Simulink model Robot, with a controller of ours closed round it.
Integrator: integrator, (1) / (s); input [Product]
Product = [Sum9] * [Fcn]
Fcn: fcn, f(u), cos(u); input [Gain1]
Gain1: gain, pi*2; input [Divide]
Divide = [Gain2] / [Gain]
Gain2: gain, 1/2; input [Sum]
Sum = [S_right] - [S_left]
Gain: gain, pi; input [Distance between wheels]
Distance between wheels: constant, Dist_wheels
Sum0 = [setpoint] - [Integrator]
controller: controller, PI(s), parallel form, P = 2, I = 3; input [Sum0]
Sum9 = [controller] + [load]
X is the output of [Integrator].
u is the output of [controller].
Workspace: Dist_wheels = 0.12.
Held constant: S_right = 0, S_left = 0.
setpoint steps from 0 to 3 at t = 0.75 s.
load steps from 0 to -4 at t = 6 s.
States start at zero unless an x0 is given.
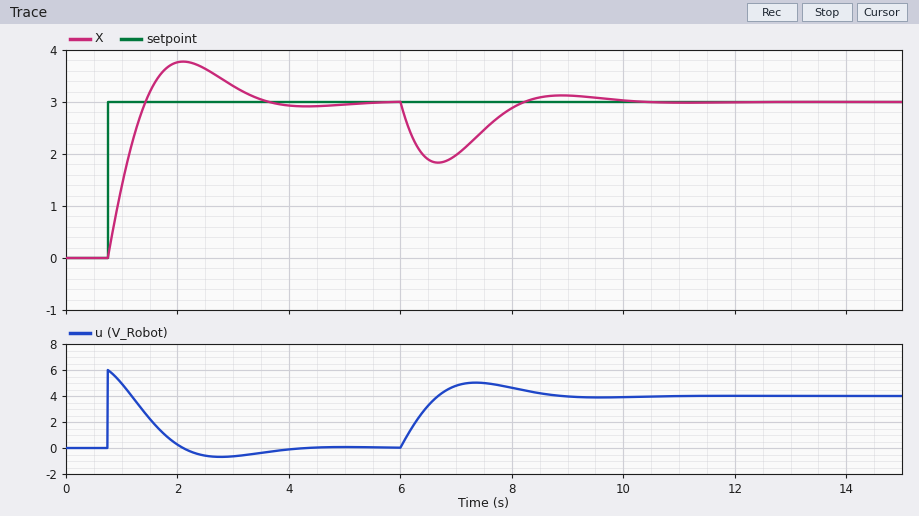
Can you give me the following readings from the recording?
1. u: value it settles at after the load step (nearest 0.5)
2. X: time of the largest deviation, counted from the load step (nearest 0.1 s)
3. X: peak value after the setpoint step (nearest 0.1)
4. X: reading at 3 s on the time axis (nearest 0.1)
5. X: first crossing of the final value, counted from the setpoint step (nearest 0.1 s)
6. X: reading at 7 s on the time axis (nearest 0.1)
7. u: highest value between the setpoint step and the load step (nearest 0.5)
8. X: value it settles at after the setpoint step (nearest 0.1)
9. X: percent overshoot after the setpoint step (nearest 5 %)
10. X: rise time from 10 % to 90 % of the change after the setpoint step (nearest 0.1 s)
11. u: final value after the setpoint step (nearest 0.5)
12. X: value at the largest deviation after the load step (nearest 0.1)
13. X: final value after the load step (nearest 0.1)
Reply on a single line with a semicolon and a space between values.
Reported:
4.0; 0.7 s; 3.8; 3.3; 0.7 s; 2.0; 6.0; 3.0; 25 %; 0.5 s; 0.0; 1.8; 3.0
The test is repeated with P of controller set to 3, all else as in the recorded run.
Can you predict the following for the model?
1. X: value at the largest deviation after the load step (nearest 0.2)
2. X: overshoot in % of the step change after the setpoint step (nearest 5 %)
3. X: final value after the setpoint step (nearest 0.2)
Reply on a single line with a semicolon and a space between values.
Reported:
2.0; 15 %; 3.0
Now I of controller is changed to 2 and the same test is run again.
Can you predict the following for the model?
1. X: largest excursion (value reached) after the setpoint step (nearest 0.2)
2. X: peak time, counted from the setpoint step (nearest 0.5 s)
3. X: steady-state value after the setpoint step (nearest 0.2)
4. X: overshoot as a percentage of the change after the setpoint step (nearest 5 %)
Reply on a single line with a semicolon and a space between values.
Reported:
3.6; 1.5 s; 3.0; 20 %
